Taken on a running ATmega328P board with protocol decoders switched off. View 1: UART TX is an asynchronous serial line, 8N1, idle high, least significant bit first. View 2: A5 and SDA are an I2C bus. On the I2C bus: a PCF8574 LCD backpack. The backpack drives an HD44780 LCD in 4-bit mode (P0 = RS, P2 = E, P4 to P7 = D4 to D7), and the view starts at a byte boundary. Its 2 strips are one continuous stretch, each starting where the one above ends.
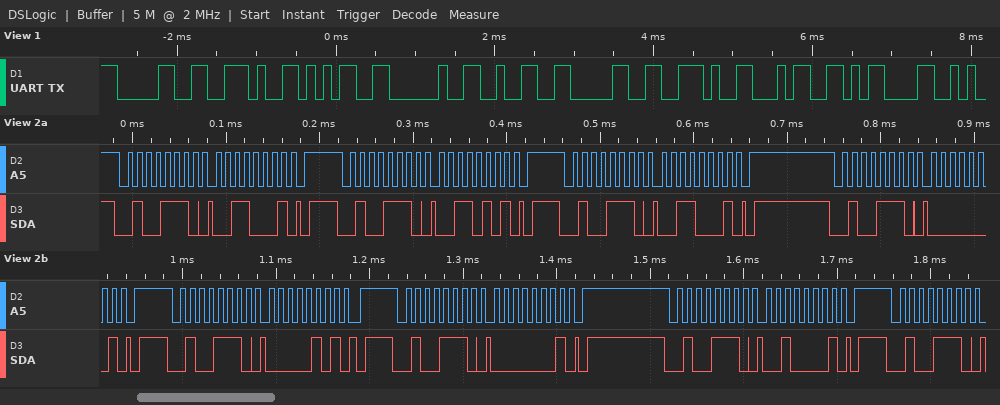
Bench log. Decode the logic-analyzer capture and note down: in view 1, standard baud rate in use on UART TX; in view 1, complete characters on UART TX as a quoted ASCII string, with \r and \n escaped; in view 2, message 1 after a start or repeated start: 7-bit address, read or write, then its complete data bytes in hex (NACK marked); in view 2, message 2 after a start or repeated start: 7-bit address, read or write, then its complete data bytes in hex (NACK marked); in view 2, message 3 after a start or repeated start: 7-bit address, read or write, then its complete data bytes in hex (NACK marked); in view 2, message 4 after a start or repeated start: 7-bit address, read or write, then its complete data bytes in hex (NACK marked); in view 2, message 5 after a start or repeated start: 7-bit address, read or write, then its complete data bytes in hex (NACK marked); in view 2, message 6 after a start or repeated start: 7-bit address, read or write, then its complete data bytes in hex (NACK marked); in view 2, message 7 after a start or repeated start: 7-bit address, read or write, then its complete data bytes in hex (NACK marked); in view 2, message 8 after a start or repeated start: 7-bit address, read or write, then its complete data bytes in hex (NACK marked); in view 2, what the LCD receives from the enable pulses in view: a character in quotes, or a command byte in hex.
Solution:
9600 baud
"0.5 20.4\r"
0x27 write: 31
0x27 write: 35
0x27 write: 31
0x27 write: 01
0x27 write: 05
0x27 write: 01
0x27 write: 21
0x27 write
'0'
